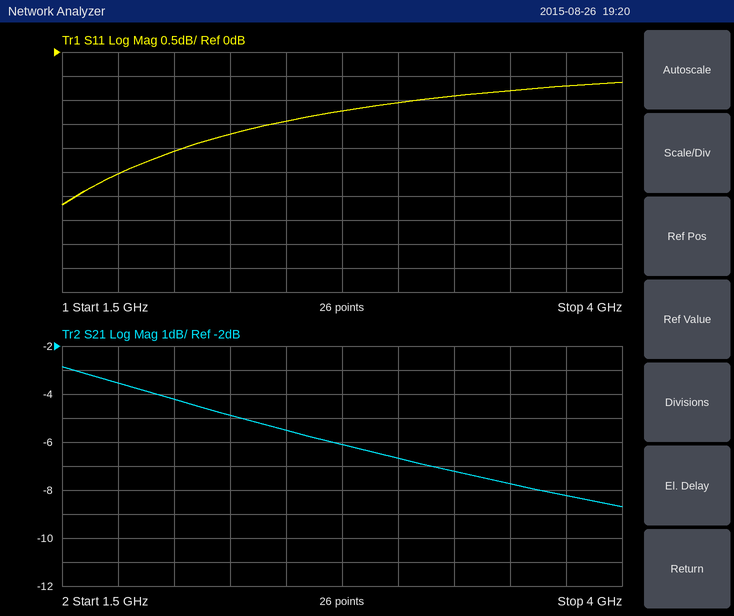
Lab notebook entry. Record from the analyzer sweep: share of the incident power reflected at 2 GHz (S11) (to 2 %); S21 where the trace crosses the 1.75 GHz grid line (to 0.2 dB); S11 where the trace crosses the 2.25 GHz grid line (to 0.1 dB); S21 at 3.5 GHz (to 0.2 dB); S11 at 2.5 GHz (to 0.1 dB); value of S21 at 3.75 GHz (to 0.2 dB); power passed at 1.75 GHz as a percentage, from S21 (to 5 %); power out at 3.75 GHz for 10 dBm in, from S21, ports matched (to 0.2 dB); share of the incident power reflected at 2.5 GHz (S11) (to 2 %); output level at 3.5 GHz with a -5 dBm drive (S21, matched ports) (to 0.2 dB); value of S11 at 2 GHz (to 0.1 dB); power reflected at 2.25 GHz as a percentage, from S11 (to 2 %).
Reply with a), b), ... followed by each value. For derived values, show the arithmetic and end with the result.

a) 10^(-2.1/10) ≈ 62 %
b) -3.6 dB
c) -1.7 dB
d) -7.8 dB
e) -1.4 dB
f) -8.2 dB
g) 10^(-3.6/10) ≈ 43.7 %, so 45 % to the nearest 5 %
h) 10 dBm + (-8.2 dB) = 1.8 dBm
i) 10^(-1.4/10) ≈ 72 %
j) -5 dBm + (-7.8 dB) = -12.8 dBm
k) -2.1 dB
l) 10^(-1.7/10) ≈ 68 %
